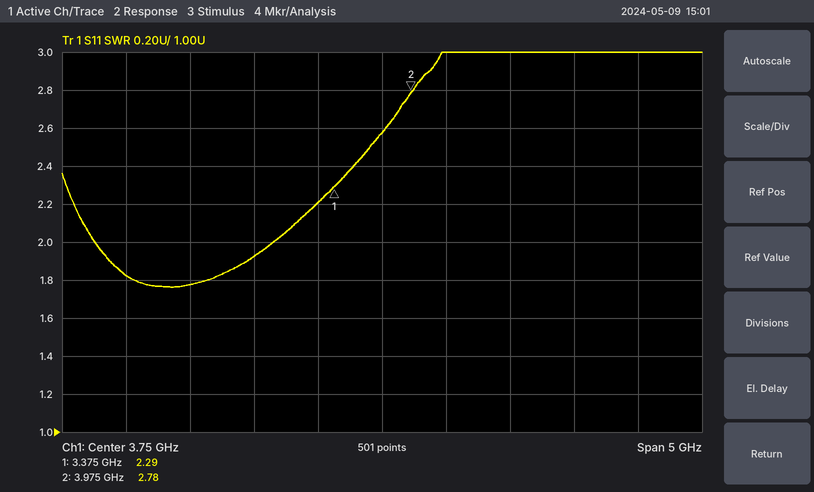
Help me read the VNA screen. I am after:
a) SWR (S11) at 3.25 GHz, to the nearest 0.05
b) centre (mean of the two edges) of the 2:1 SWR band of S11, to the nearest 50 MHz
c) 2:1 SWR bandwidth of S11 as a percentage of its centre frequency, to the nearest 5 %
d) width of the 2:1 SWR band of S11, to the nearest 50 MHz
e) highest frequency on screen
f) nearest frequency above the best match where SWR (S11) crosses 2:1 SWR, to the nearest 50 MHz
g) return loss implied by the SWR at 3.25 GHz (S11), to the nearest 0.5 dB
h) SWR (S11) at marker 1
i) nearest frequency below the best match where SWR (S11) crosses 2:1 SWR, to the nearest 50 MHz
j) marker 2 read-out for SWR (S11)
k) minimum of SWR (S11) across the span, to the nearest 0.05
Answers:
2.20
2.20 GHz
65 %
1.40 GHz
6.25 GHz
2.90 GHz
8.5 dB
2.29
1.50 GHz
2.78
1.75
